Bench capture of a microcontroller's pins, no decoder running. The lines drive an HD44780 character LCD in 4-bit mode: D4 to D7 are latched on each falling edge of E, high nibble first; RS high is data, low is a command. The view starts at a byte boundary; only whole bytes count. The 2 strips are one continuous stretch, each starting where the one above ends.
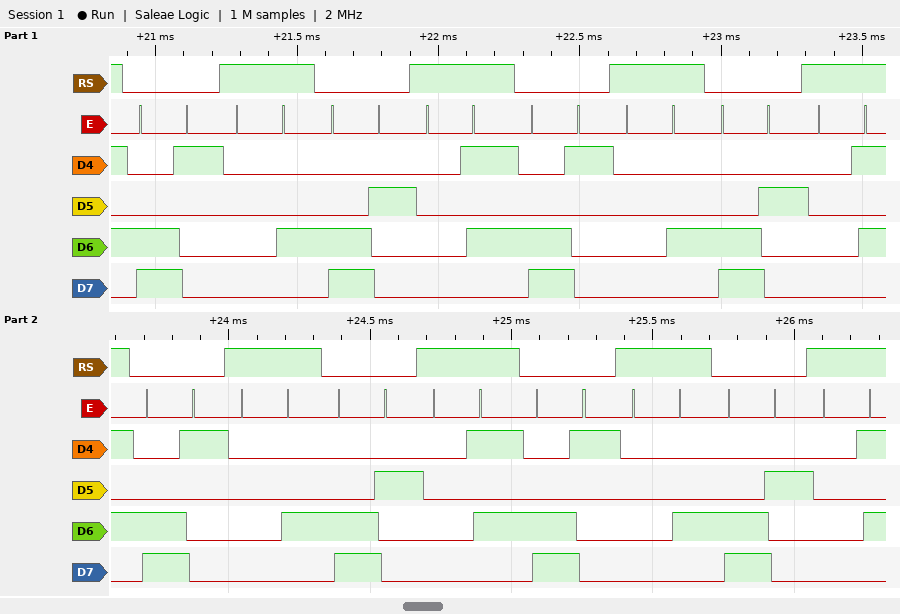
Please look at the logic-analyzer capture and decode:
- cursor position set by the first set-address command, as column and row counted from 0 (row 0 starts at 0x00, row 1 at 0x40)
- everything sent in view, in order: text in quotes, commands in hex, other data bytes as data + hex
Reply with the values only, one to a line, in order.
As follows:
column 1, row 1
0xC1 data 04 0xC2 data 05 0xC1 data 04 0xC2 data 05 0xC1 data 04 0xC2 data 05 0xC1 data 04 0xC2 data 05
